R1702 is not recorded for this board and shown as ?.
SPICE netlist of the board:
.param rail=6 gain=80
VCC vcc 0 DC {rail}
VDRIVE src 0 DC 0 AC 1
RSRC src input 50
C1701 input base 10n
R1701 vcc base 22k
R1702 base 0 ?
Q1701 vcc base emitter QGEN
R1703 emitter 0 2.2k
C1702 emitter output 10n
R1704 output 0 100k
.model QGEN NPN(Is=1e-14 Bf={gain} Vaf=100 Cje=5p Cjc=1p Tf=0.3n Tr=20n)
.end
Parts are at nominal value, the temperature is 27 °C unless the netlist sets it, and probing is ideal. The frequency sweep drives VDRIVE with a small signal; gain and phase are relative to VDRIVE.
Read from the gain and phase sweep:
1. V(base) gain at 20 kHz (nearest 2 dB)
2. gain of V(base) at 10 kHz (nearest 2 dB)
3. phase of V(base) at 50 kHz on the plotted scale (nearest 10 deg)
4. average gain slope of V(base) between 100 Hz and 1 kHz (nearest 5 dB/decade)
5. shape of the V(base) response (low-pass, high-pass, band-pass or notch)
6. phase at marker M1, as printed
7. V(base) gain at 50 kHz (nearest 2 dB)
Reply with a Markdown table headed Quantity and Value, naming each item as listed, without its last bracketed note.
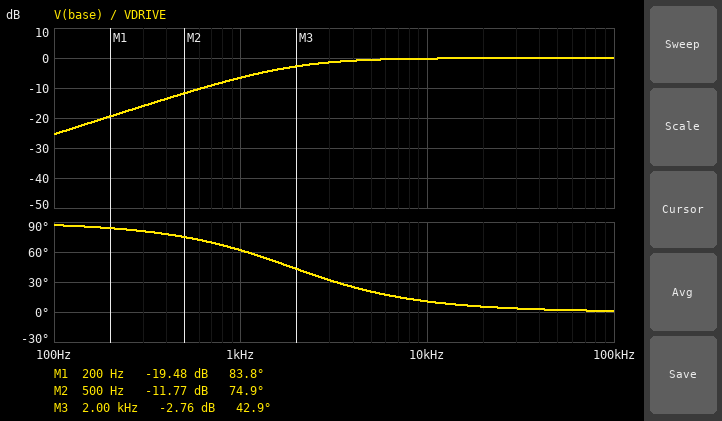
| Quantity | Value |
|---|---|
| V(base) gain at 20 kHz | 0 dB |
| gain of V(base) at 10 kHz | 0 dB |
| phase of V(base) at 50 kHz on the plotted scale | 0 deg |
| average gain slope of V(base) between 100 Hz and 1 kHz | 20 dB/decade |
| shape of the V(base) response | high-pass |
| phase at marker M1, as printed | 83.8 deg |
| V(base) gain at 50 kHz | 0 dB |
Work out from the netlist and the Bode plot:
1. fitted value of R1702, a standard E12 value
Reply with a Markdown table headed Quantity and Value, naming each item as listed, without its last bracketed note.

| Quantity | Value |
|---|---|
| fitted value of R1702, a standard E12 value | 15 kΩ |
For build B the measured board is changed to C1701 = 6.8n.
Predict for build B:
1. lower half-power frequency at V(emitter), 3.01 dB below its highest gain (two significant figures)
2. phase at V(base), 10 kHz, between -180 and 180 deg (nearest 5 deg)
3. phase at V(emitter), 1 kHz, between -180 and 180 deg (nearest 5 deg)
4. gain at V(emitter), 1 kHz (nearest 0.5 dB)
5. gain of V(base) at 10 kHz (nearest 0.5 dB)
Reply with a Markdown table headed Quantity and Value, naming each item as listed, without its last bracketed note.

| Quantity | Value |
|---|---|
| lower half-power frequency at V(emitter), 3.01 dB below its highest gain | 2.7 kHz |
| phase at V(base), 10 kHz, between -180 and 180 deg | 15 deg |
| phase at V(emitter), 1 kHz, between -180 and 180 deg | 70 deg |
| gain at V(emitter), 1 kHz | -9.5 dB |
| gain of V(base) at 10 kHz | -0.5 dB |
